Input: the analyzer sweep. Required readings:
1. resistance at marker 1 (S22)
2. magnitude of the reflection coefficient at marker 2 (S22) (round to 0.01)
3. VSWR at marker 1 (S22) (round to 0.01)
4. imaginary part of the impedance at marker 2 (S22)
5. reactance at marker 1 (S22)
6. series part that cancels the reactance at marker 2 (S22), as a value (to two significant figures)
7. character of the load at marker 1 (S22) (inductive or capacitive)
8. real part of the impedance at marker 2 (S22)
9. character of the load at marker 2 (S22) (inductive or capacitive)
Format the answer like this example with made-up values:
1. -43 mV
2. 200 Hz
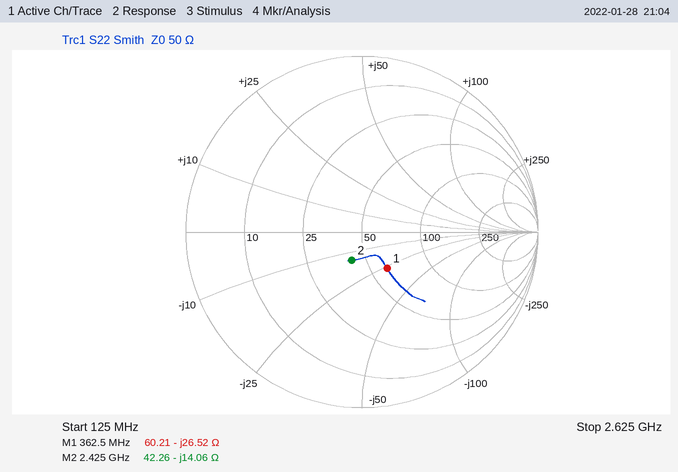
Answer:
1. 60.21 Ω
2. 0.17
3. 1.67
4. -14.06 Ω
5. -26.52 Ω
6. 920 pH
7. capacitive
8. 42.26 Ω
9. capacitive
